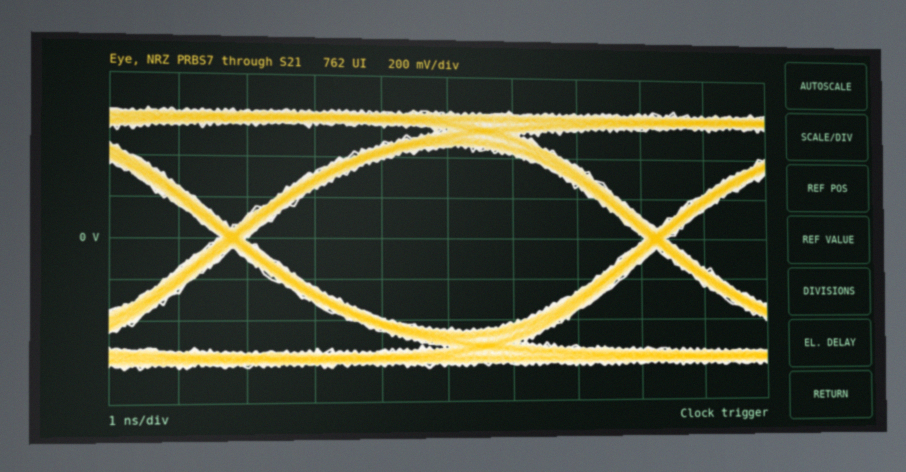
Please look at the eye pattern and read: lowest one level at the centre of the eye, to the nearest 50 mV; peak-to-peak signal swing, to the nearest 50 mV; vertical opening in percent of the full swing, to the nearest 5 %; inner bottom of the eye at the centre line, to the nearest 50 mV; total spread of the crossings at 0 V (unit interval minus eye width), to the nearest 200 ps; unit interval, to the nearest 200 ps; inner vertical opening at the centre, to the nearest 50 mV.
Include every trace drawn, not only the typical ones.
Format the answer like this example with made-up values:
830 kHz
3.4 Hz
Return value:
450 mV
1.30 V
70 %
-450 mV
400 ps
6.4 ns
900 mV
